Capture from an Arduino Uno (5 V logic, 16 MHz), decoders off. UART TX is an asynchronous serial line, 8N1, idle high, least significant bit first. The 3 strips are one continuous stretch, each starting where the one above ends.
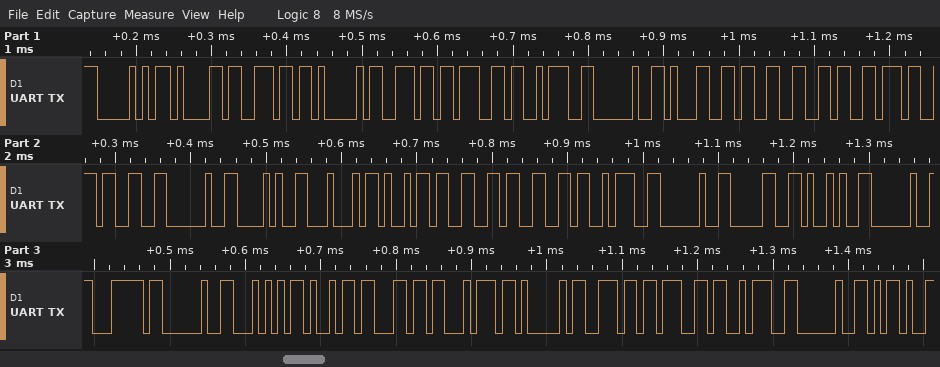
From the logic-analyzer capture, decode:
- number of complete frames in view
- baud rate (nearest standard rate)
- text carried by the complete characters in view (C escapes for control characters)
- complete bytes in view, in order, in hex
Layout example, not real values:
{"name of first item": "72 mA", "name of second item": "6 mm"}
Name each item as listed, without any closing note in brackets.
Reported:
{"number of complete frames in view": "36", "baud rate": "115200 baud", "text carried by the complete characters in view": "\"PanAng: 13673 (Diff: 0) | TiltAng: -\"", "complete bytes in view, in order, in hex": "50 61 6E 41 6E 67 3A 20 31 33 36 37 33 20 28 44 69 66 66 3A 20 30 29 20 7C 20 54 69 6C 74 41 6E 67 3A 20 2D"}
